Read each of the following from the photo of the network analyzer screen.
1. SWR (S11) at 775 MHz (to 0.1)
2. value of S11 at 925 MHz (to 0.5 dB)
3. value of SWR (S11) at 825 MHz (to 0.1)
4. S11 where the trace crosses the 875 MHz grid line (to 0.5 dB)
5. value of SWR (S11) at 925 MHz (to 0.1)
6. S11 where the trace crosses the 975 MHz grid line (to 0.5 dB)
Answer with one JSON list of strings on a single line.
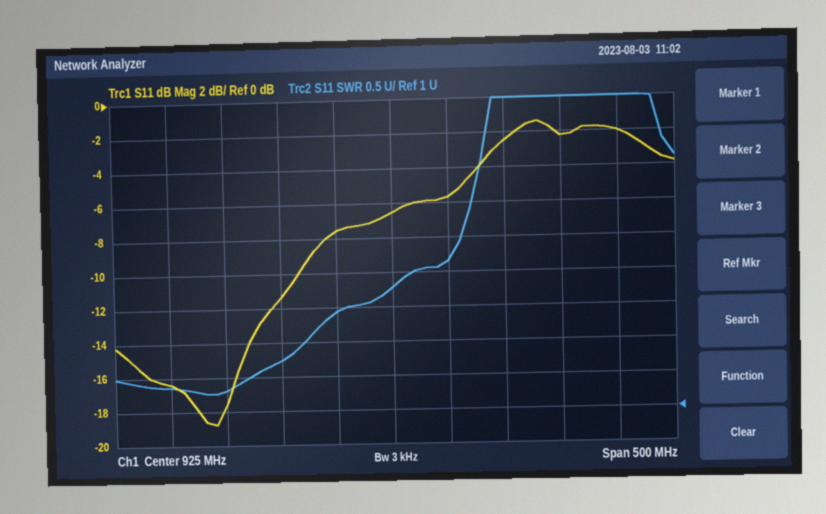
["1.3", "-6.5 dB", "1.7", "-7.5 dB", "2.8", "-5.5 dB"]
